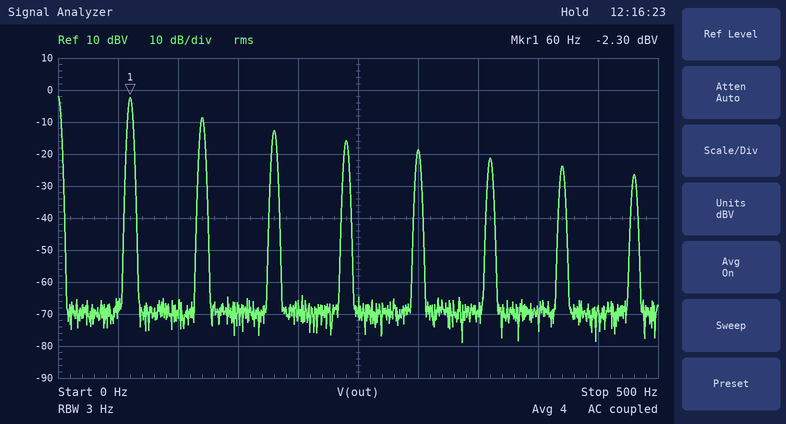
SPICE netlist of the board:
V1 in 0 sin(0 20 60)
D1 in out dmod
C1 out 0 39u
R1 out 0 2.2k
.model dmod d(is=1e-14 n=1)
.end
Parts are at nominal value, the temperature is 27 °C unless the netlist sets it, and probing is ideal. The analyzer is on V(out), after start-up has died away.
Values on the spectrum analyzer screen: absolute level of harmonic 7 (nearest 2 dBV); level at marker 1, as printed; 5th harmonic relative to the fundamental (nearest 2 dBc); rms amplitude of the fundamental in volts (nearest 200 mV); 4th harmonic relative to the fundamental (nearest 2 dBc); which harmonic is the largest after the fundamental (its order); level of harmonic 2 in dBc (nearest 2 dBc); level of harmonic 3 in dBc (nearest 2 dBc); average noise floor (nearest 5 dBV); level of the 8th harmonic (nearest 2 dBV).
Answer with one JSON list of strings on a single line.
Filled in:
["-24 dBV", "-2.30 dBV", "-16 dBc", "800 mV", "-14 dBc", "2", "-6 dBc", "-10 dBc", "-70 dBV", "-26 dBV"]
